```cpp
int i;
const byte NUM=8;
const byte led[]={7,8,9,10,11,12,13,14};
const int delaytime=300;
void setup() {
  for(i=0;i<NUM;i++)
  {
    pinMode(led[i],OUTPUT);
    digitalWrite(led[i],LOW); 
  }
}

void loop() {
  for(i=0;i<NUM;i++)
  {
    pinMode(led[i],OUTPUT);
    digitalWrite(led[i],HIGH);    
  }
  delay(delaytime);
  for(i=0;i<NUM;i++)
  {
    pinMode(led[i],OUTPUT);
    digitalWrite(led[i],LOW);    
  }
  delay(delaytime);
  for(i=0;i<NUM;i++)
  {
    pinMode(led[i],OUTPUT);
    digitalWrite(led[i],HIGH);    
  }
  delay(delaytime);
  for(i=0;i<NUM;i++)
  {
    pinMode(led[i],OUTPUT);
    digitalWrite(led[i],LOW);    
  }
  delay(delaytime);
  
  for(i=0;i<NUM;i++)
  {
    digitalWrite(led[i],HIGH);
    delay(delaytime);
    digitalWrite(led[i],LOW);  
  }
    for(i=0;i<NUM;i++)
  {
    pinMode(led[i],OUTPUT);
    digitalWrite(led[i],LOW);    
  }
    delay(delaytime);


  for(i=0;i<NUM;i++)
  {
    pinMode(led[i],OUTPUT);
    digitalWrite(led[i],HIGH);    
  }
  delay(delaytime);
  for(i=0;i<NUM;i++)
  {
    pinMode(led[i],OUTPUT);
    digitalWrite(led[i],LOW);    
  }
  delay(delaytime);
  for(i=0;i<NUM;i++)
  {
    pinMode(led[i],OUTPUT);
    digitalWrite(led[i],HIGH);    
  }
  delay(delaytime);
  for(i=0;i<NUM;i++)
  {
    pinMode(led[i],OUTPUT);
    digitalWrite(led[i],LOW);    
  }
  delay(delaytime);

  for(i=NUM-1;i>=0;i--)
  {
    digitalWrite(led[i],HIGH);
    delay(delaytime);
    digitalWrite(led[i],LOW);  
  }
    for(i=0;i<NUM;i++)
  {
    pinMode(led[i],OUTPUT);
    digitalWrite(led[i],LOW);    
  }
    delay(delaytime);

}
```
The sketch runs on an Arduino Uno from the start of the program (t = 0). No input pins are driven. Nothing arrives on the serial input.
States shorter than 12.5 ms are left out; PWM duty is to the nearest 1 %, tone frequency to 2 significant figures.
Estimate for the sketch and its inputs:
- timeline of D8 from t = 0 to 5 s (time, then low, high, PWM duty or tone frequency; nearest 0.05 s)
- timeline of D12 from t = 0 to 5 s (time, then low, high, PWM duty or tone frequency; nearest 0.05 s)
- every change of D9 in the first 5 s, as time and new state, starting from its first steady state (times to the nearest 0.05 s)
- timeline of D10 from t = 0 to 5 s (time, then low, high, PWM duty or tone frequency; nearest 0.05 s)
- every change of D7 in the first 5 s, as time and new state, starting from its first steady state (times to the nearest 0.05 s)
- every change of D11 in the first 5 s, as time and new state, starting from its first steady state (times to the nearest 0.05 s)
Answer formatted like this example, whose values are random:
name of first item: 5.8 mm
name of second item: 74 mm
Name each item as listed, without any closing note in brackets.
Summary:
timeline of D8 from t = 0 to 5 s: 0 s high; 0.3 s low; 0.6 s high; 0.9 s low; 1.5 s high; 1.8 s low; 3.9 s high; 4.2 s low; 4.5 s high; 4.8 s low
timeline of D12 from t = 0 to 5 s: 0 s high; 0.3 s low; 0.6 s high; 0.9 s low; 2.7 s high; 3 s low; 3.9 s high; 4.2 s low; 4.5 s high; 4.8 s low
every change of D9 in the first 5 s, as time and new state, starting from its first steady state: 0 s high; 0.3 s low; 0.6 s high; 0.9 s low; 1.8 s high; 2.1 s low; 3.9 s high; 4.2 s low; 4.5 s high; 4.8 s low
timeline of D10 from t = 0 to 5 s: 0 s high; 0.3 s low; 0.6 s high; 0.9 s low; 2.1 s high; 2.4 s low; 3.9 s high; 4.2 s low; 4.5 s high; 4.8 s low
every change of D7 in the first 5 s, as time and new state, starting from its first steady state: 0 s high; 0.3 s low; 0.6 s high; 0.9 s low; 1.2 s high; 1.5 s low; 3.9 s high; 4.2 s low; 4.5 s high; 4.8 s low
every change of D11 in the first 5 s, as time and new state, starting from its first steady state: 0 s high; 0.3 s low; 0.6 s high; 0.9 s low; 2.4 s high; 2.7 s low; 3.9 s high; 4.2 s low; 4.5 s high; 4.8 s low
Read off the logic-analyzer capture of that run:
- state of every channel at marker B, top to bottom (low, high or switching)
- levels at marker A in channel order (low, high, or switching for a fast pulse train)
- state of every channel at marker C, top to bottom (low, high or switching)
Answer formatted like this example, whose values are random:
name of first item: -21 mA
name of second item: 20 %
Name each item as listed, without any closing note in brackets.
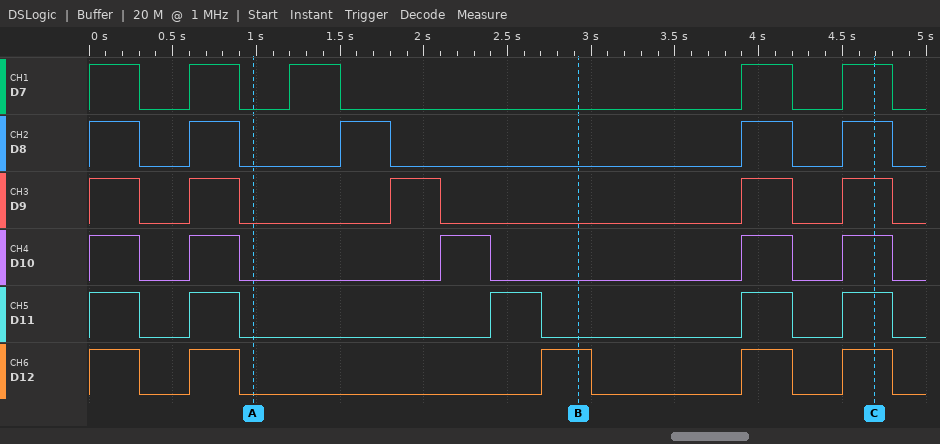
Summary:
state of every channel at marker B, top to bottom: D7 low, D8 low, D9 low, D10 low, D11 low, D12 high
levels at marker A in channel order: D7 low, D8 low, D9 low, D10 low, D11 low, D12 low
state of every channel at marker C, top to bottom: D7 high, D8 high, D9 high, D10 high, D11 high, D12 high
